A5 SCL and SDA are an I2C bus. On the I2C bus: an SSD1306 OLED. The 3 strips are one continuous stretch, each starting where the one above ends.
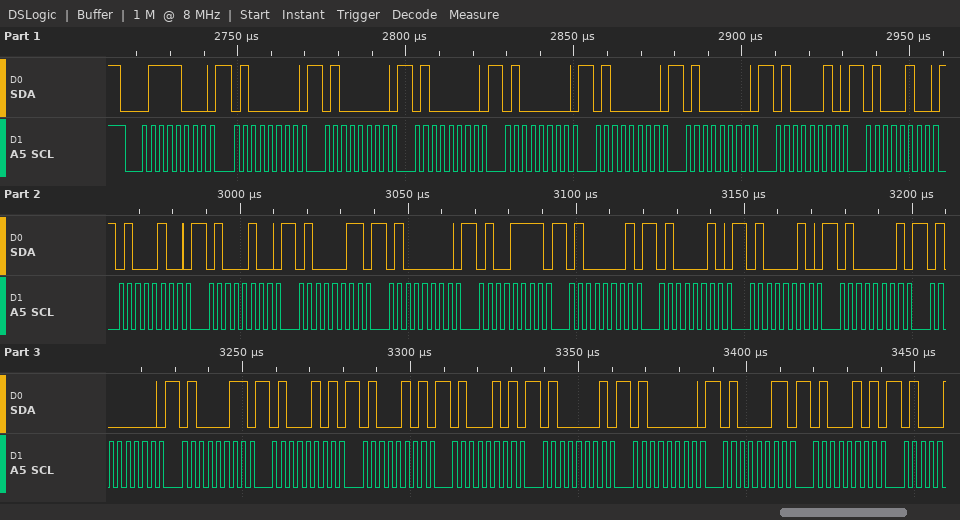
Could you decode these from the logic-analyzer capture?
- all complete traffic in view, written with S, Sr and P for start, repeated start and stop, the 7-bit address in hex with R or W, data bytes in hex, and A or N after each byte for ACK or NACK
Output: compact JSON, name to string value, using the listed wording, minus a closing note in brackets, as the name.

{"all complete traffic in view, written with S, Sr and P for start, repeated start and stop, the 7-bit address in hex with R or W, data bytes in hex, and A or N after each byte for ACK or NACK": "S 3CW A 40 A 40 A 40 A 40 A 40 A 40 A 42 A 44 A 44 A 44 A 43 A 40 A 4F A 41 A 42 A 42 A 41 A 40 A 43 A 45 A 45 A 45 A 41 A 40 A 43 A 45 A"}
